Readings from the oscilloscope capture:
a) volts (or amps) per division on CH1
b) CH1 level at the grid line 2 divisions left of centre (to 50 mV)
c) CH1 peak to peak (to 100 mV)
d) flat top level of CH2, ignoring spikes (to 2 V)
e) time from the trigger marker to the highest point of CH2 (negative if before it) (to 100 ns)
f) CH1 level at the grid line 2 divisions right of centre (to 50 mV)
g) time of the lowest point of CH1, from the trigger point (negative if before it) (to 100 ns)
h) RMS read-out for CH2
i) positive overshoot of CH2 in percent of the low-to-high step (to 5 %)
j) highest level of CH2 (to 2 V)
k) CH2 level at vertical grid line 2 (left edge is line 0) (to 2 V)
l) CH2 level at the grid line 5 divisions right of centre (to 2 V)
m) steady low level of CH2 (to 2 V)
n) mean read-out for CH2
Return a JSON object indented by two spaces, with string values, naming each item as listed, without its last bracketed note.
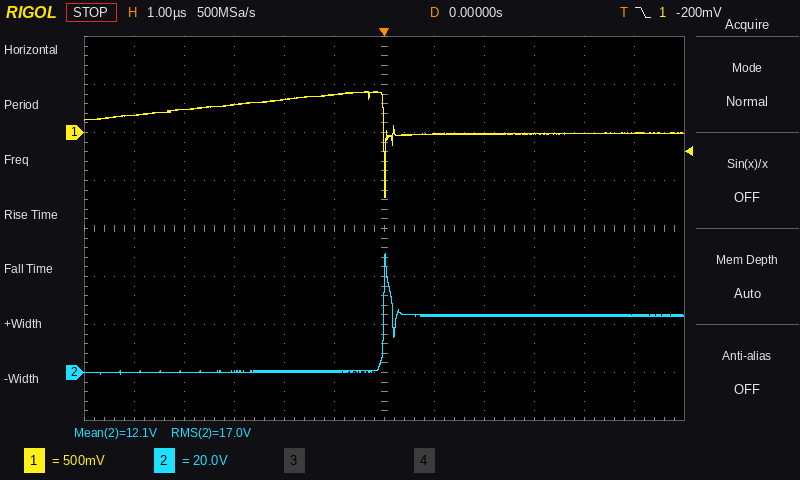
{
  "volts (or amps) per division on CH1": "500 mV",
  "CH1 level at the grid line 2 divisions left of centre": "350 mV",
  "CH1 peak to peak": "1.10 V",
  "flat top level of CH2, ignoring spikes": "24 V",
  "time from the trigger marker to the highest point of CH2 (negative if before it)": "0.0 µs",
  "CH1 level at the grid line 2 divisions right of centre": "0 mV",
  "time of the lowest point of CH1, from the trigger point (negative if before it)": "0.0 µs",
  "RMS read-out for CH2": "17.0 V",
  "positive overshoot of CH2 in percent of the low-to-high step": "110 %",
  "highest level of CH2": "50 V",
  "CH2 level at vertical grid line 2 (left edge is line 0)": "0 V",
  "CH2 level at the grid line 5 divisions right of centre": "24 V",
  "steady low level of CH2": "0 V",
  "mean read-out for CH2": "12.1 V"
}
